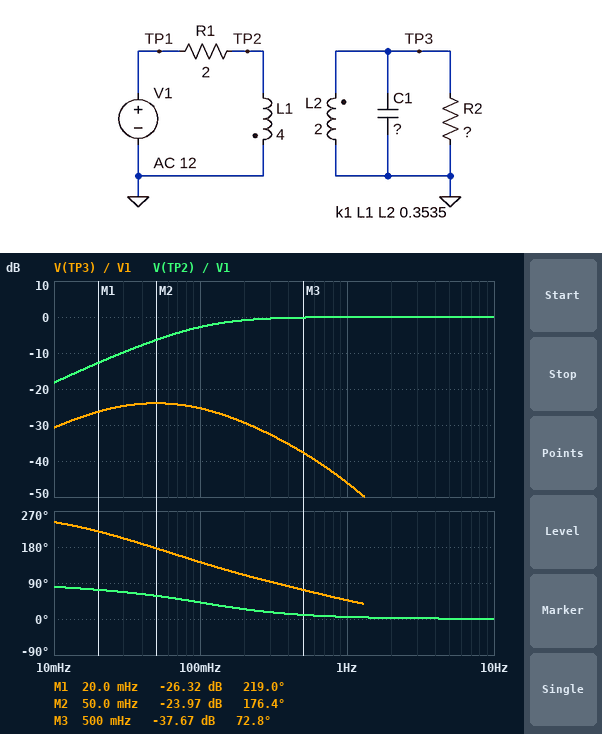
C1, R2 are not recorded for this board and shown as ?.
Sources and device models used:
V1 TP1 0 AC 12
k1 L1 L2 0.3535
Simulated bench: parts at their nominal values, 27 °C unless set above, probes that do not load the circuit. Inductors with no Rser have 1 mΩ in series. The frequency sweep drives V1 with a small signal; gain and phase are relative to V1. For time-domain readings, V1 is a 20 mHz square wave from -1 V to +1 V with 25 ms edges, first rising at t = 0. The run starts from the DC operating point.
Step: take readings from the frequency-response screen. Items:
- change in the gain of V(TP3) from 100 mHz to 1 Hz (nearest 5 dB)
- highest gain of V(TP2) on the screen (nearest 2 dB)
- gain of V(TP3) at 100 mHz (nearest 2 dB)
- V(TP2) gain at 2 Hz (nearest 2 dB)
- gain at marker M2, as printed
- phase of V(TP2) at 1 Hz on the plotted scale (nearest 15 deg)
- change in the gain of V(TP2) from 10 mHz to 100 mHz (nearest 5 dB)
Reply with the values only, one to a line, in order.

-20 dB
0 dB
-26 dB
0 dB
-23.97 dB
0 deg
15 dB
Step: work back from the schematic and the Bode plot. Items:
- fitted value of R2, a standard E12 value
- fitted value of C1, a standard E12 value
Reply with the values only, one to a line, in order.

0.33 Ω
560 mF
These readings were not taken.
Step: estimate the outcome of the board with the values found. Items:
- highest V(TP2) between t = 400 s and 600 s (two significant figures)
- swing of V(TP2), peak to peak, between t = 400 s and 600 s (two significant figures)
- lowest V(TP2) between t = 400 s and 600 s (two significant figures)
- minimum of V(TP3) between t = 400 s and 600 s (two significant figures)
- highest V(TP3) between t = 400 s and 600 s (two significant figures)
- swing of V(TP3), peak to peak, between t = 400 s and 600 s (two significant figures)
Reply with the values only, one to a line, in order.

2.0 V
4.0 V
-2.0 V
-97 mV
97 mV
190 mV
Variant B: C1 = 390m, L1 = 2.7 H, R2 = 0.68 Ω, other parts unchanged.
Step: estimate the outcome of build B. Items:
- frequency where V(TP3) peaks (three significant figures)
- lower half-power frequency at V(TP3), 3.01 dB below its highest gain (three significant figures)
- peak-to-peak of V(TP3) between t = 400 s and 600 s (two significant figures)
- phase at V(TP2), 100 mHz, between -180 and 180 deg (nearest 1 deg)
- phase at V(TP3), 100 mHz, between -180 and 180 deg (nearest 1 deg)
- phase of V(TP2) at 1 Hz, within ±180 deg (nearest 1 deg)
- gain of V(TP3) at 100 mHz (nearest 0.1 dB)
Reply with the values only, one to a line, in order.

88.1 mHz
33.7 mHz
310 mV
50 deg
165 deg
8 deg
-19.9 dB
